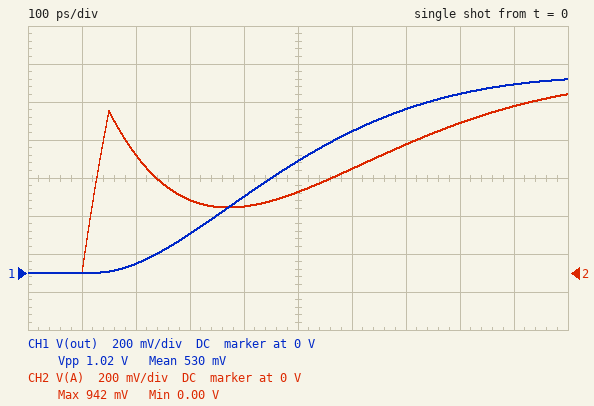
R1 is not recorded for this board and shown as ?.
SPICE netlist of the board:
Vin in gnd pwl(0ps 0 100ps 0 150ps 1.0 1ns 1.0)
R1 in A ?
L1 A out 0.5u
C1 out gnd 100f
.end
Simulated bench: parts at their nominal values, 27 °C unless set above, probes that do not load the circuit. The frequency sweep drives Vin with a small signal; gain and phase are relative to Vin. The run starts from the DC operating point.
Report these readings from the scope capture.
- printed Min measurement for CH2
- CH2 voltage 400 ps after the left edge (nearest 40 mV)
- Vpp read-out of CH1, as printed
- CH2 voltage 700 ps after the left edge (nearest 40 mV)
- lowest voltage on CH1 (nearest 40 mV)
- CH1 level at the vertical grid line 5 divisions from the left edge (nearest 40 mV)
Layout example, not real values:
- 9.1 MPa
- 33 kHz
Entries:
- 0.00 V
- 360 mV
- 1.02 V
- 680 mV
- 0 V
- 600 mV
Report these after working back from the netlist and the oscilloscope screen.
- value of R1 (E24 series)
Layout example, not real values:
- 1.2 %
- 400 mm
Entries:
- 3.3 kΩ
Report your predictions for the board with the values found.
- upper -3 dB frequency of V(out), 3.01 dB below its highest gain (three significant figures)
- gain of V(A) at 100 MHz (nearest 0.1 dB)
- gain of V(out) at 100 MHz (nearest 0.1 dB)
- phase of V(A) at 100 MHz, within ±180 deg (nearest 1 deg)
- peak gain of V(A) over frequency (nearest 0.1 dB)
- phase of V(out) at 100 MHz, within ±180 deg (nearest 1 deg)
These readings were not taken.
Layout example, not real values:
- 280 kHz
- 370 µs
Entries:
- 681 MHz
- -0.2 dB
- 0 dB
- -12 deg
- 0 dB
- -12 deg
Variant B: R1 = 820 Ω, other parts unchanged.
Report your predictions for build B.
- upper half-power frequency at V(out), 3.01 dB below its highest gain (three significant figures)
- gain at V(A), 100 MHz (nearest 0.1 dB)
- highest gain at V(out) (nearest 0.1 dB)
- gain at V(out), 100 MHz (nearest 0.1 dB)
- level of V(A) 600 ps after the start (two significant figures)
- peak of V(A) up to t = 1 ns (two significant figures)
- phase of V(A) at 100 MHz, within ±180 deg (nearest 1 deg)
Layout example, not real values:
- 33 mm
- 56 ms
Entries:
- 809 MHz
- 0 dB
- 8.9 dB
- 0.2 dB
- 780 mV
- 1.1 V
- -3 deg
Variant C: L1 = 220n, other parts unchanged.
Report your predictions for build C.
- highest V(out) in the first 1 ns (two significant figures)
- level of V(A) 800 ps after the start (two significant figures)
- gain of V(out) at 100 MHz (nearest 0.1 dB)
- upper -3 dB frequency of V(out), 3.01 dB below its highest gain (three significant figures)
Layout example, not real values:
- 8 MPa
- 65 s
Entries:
- 960 mV
- 870 mV
- -0.1 dB
- 595 MHz
